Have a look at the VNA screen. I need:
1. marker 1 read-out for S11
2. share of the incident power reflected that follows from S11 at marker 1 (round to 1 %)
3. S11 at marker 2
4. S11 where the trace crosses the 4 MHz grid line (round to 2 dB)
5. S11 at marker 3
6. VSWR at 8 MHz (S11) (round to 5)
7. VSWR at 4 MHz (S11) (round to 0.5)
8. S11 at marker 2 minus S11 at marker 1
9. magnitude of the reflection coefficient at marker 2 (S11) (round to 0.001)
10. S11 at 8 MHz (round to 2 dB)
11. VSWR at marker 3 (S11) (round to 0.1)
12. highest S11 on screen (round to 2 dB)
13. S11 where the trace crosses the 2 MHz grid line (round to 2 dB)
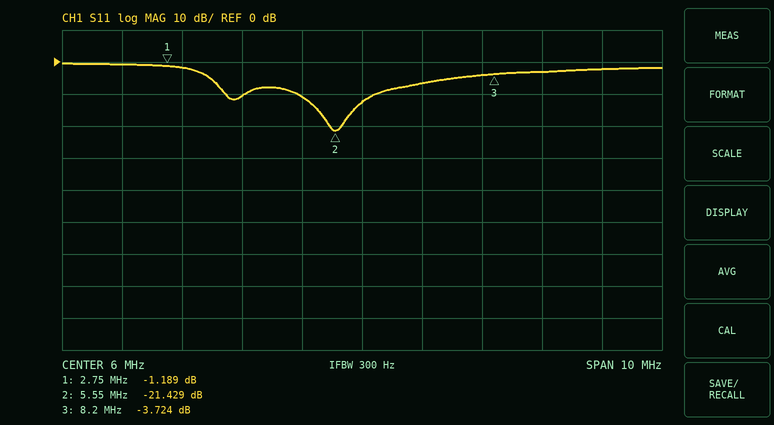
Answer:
-1.189 dB
76 %
-21.429 dB
-10 dB
-3.724 dB
5
2.0
-20.240 dB
0.085
-4 dB
4.7
0 dB
0 dB
